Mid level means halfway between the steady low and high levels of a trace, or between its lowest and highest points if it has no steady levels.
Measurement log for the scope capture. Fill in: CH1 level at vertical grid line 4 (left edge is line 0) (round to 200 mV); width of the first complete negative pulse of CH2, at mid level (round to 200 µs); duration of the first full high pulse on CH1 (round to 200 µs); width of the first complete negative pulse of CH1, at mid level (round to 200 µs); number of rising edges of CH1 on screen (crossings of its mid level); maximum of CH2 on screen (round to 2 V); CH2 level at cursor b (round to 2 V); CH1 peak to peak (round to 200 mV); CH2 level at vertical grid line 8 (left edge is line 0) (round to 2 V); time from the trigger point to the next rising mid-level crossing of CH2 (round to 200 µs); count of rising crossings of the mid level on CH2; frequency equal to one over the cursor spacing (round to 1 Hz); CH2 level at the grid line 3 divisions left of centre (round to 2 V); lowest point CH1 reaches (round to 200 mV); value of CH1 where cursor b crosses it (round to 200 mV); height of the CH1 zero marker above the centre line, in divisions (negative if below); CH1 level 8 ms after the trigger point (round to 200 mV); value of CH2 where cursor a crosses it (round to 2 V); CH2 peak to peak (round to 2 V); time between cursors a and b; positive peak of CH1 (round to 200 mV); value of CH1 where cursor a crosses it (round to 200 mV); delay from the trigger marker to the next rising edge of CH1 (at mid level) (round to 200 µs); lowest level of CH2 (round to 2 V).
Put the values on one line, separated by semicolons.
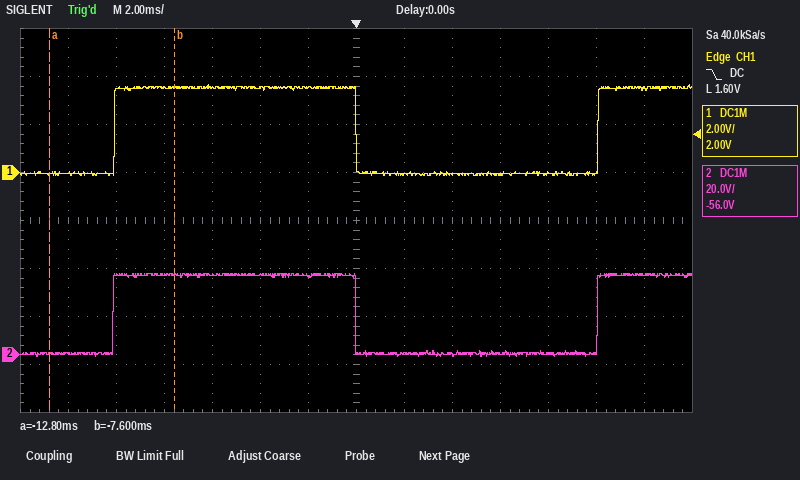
3.6 V; 10.0 ms; 10.0 ms; 10.0 ms; 2; 34 V; 34 V; 3.8 V; 0 V; 10.0 ms; 2; 192 Hz; 34 V; -200 mV; 3.6 V; +1.0 div; 0.0 V; 0 V; 34 V; 5.2 ms; 3.6 V; 0.0 V; 10.0 ms; 0 V
